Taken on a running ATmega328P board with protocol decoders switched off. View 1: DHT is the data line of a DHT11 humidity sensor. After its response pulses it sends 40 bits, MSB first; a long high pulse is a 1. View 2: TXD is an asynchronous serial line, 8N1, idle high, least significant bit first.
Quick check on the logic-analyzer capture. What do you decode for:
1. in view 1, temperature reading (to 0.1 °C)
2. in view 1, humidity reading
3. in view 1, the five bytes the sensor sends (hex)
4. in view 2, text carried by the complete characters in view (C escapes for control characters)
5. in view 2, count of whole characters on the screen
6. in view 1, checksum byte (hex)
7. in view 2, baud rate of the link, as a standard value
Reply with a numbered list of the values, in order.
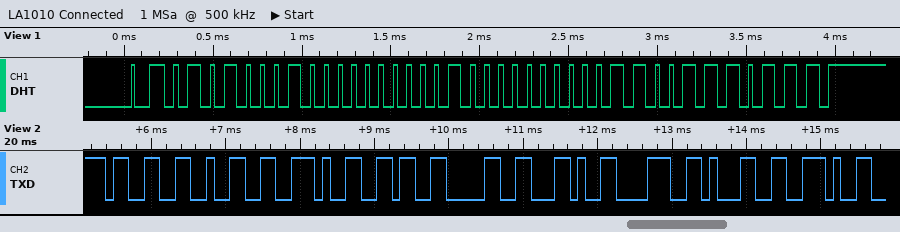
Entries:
1. 32.6 °C
2. 81 %
3. 51 00 20 06 77
4. "32.60,81."
5. 9
6. 0x77
7. 9600 baud
